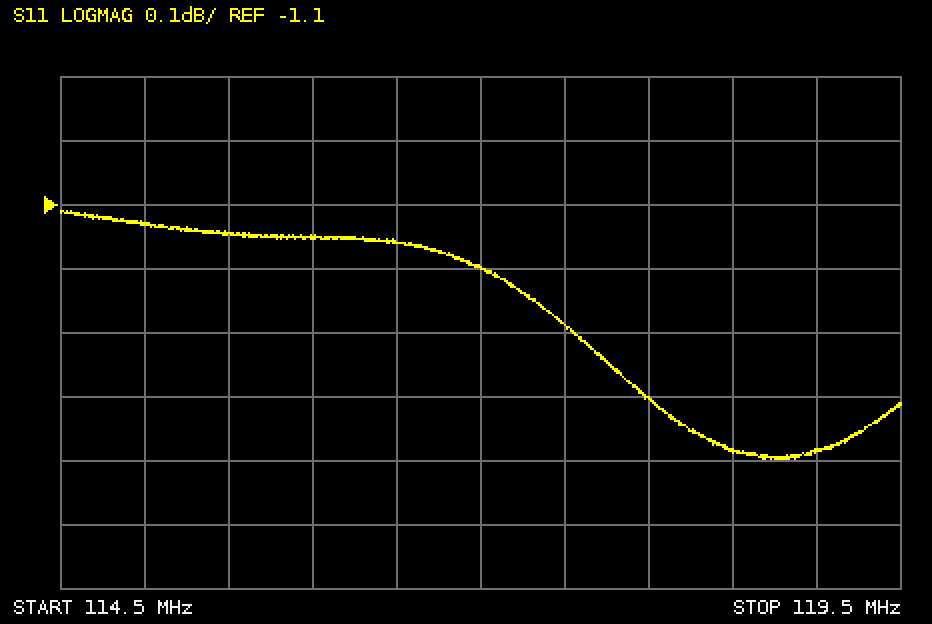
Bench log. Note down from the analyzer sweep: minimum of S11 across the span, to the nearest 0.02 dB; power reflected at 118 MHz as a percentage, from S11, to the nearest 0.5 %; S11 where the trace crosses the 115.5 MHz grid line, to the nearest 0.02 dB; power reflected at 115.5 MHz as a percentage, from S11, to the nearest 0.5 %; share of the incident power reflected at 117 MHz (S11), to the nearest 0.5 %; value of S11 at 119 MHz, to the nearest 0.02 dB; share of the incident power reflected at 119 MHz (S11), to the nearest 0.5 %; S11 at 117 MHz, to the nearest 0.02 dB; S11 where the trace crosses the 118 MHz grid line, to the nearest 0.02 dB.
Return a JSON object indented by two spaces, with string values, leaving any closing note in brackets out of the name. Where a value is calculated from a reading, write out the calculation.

{
  "minimum of S11 across the span, to the nearest 0.02 dB": "-1.50 dB",
  "power reflected at 118 MHz as a percentage, from S11, to the nearest 0.5 %": "10^(-1.4/10) ≈ 72.4 %, so 72.5 % to the nearest 0.5 %",
  "S11 where the trace crosses the 115.5 MHz grid line, to the nearest 0.02 dB": "-1.14 dB",
  "power reflected at 115.5 MHz as a percentage, from S11, to the nearest 0.5 %": "10^(-1.14/10) ≈ 76.9 %, so 77.0 % to the nearest 0.5 %",
  "share of the incident power reflected at 117 MHz (S11), to the nearest 0.5 %": "10^(-1.2/10) ≈ 75.9 %, so 76.0 % to the nearest 0.5 %",
  "value of S11 at 119 MHz, to the nearest 0.02 dB": "-1.48 dB",
  "share of the incident power reflected at 119 MHz (S11), to the nearest 0.5 %": "10^(-1.48/10) ≈ 71.1 %, so 71.0 % to the nearest 0.5 %",
  "S11 at 117 MHz, to the nearest 0.02 dB": "-1.20 dB",
  "S11 where the trace crosses the 118 MHz grid line, to the nearest 0.02 dB": "-1.40 dB"
}
